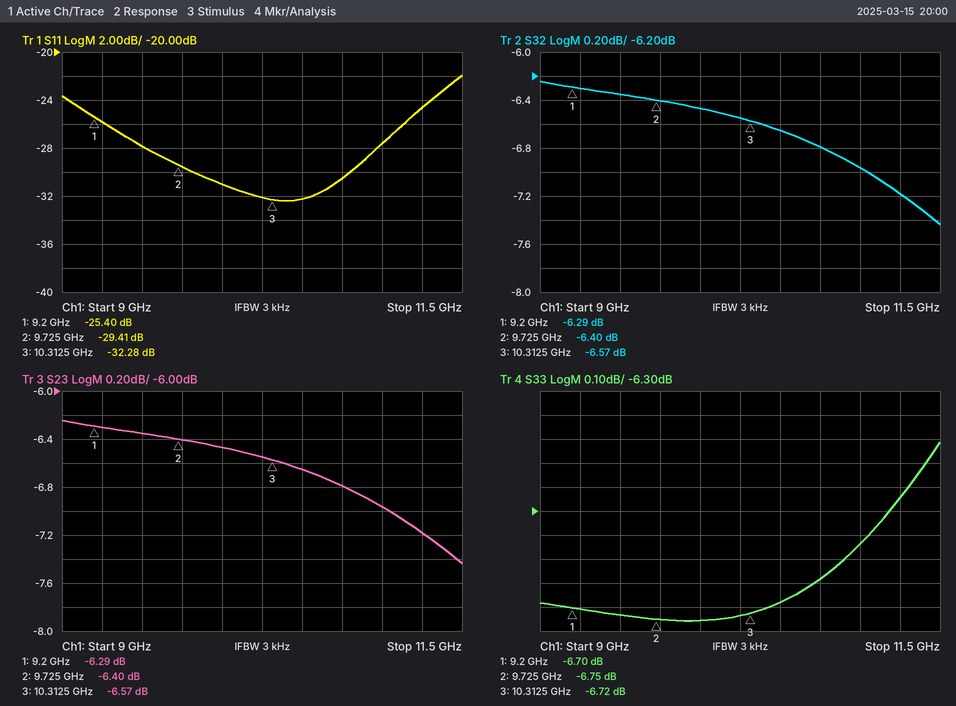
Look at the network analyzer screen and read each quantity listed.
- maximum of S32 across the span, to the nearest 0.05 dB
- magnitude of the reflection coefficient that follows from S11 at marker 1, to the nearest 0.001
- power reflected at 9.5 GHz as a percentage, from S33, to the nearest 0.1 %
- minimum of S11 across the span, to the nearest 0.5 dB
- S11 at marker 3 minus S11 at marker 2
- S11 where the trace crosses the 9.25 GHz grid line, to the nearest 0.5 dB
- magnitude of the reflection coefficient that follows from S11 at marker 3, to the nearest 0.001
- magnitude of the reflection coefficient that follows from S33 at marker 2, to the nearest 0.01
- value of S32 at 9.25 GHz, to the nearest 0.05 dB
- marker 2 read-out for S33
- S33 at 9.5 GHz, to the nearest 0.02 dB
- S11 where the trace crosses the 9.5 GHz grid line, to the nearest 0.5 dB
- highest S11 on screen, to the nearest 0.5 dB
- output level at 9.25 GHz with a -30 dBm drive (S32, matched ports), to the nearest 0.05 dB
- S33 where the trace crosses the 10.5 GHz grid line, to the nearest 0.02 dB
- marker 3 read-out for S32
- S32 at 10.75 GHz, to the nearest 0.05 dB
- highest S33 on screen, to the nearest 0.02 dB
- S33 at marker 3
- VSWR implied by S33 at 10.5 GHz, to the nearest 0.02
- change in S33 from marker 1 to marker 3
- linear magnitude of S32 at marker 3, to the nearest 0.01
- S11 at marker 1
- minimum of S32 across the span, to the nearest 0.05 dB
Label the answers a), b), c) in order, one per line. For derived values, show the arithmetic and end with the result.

a) -6.25 dB
b) 10^(-25.4/20) ≈ 0.054
c) 10^(-6.74/10) ≈ 21.2 %
d) -32.5 dB
e) -32.28 − (-29.41) = -2.87 dB
f) -26.0 dB
g) 10^(-32.28/20) ≈ 0.024
h) 10^(-6.75/20) ≈ 0.46
i) -6.30 dB
j) -6.75 dB
k) -6.74 dB
l) -28.0 dB
m) -22.0 dB
n) -30 dBm + (-6.30 dB) = -36.30 dBm
o) -6.68 dB
p) -6.57 dB
q) -6.80 dB
r) -6.02 dB
s) -6.72 dB
t) |Γ| = 10^(-6.68/20) = 0.4634; VSWR = (1 + 0.4634)/(1 − 0.4634) ≈ 2.73, so 2.72 to the nearest 0.02
u) -6.72 − (-6.7) = -0.02 dB
v) 10^(-6.57/20) ≈ 0.47
w) -25.40 dB
x) -7.45 dB
